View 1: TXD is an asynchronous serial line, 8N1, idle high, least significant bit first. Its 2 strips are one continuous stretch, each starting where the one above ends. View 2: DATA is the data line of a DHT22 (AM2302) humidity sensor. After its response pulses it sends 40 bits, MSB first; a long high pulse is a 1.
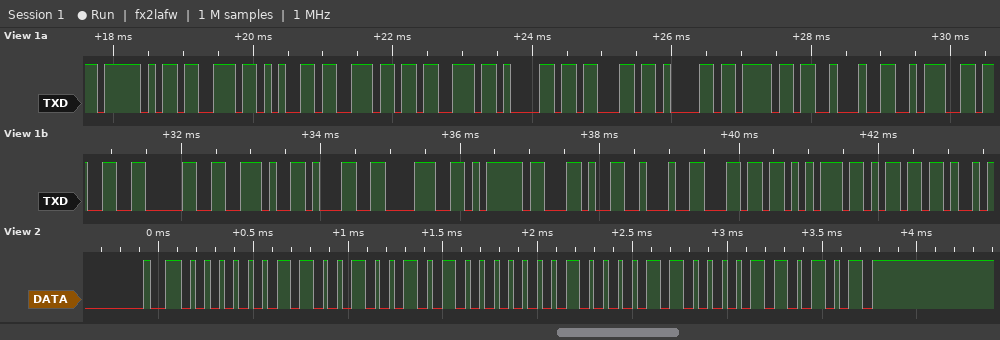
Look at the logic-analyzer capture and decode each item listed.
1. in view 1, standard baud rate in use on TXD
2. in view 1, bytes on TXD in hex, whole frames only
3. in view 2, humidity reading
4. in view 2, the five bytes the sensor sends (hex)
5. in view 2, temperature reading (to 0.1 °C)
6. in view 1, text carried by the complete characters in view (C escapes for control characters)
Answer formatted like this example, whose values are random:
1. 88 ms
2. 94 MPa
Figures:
1. 9600 baud
2. 5F 73 65 6E 73 61 63 61 6F 22 3A 33 30 2E 31 38 7D 2C 22 6C 75 6D
3. 80.5 %
4. 03 25 01 0C 35
5. 26.8 °C
6. "_sensacao\":30.18},\"lum"
